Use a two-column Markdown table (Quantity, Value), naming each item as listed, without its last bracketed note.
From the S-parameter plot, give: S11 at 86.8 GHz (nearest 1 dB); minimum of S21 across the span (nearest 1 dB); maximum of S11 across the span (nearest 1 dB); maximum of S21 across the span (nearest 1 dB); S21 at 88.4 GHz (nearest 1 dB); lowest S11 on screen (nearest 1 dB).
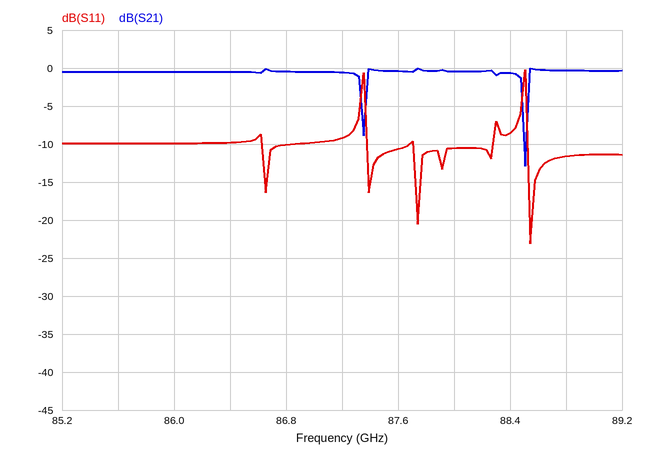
| Quantity | Value |
|---|---|
| S11 at 86.8 GHz | -10 dB |
| minimum of S21 across the span | -13 dB |
| maximum of S11 across the span | 0 dB |
| maximum of S21 across the span | 0 dB |
| S21 at 88.4 GHz | -1 dB |
| lowest S11 on screen | -23 dB |
